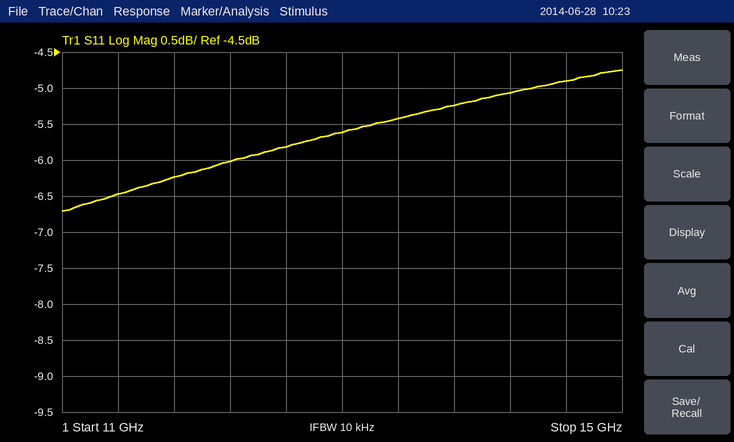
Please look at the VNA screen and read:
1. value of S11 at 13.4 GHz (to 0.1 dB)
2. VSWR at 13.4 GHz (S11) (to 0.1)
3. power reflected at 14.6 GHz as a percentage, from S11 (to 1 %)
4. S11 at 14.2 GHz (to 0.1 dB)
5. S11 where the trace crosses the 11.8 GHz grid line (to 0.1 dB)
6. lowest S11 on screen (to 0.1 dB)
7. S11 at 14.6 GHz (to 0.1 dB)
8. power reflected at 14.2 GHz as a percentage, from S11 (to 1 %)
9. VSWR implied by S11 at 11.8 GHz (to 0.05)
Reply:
-5.4 dB
3.3
32 %
-5.1 dB
-6.2 dB
-6.7 dB
-4.9 dB
31 %
2.90
